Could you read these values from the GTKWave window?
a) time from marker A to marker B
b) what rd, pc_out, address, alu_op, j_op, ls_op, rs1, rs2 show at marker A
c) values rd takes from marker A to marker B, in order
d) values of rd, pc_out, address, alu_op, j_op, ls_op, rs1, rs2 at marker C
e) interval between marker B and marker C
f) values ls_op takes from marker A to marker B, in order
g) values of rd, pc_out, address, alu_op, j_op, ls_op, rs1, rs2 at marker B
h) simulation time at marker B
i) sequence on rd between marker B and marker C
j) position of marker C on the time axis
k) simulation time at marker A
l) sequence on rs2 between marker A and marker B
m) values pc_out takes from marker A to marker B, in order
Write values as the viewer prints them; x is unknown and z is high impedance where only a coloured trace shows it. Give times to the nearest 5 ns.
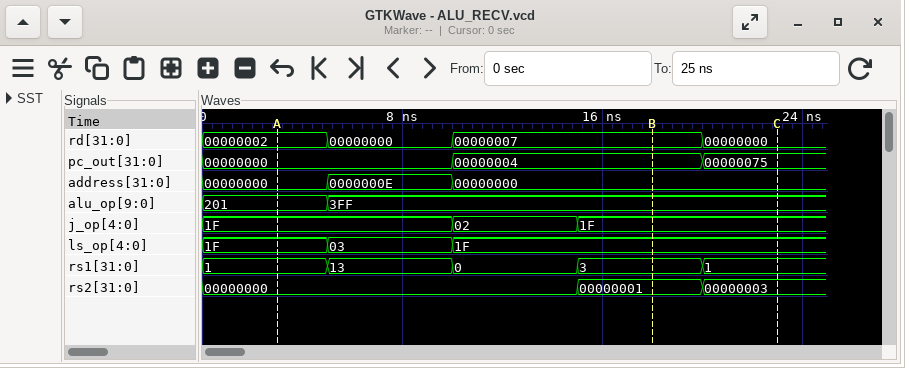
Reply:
15 ns
rd=00000002, pc_out=00000000, address=00000000, alu_op=201, j_op=1F, ls_op=1F, rs1=1, rs2=00000000
00000002, 00000000, 00000007
rd=00000000, pc_out=00000075, address=00000000, alu_op=3FF, j_op=1F, ls_op=1F, rs1=1, rs2=00000003
5 ns
1F, 03, 1F
rd=00000007, pc_out=00000004, address=00000000, alu_op=3FF, j_op=1F, ls_op=1F, rs1=3, rs2=00000001
20 ns
00000007, 00000000
25 ns
5 ns
00000000, 00000001
00000000, 00000004
